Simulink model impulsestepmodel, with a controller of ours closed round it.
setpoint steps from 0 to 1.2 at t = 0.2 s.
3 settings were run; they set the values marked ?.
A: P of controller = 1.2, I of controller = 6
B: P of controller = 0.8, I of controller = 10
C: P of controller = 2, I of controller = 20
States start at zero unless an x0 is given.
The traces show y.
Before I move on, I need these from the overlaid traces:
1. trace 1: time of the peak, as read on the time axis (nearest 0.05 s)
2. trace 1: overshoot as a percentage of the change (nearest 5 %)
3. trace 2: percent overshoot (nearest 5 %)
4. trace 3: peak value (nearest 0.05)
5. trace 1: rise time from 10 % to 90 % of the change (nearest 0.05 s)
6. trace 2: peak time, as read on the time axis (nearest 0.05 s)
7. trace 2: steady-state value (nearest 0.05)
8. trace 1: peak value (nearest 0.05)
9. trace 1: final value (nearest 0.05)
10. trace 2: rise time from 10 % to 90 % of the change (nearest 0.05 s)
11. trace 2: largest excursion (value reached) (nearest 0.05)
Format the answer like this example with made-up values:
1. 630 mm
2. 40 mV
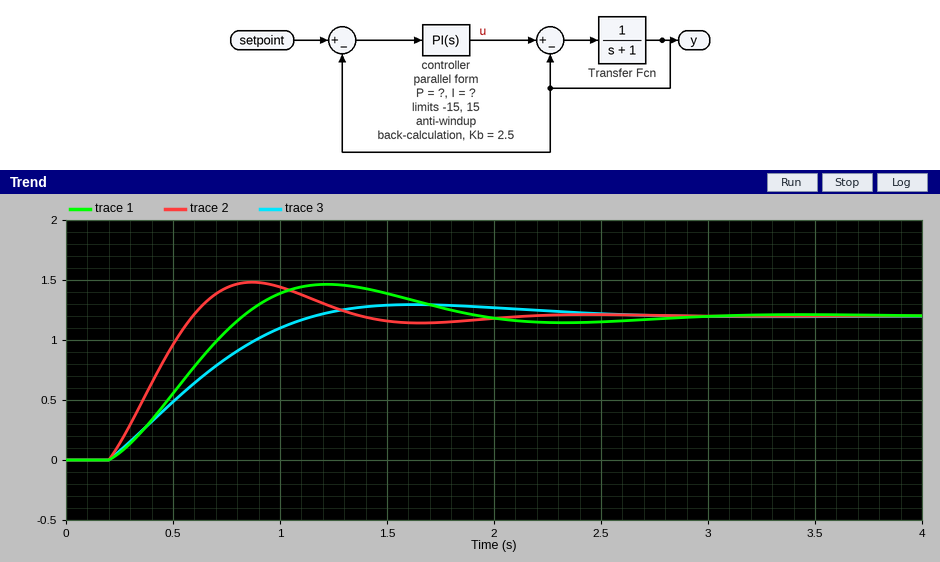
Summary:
1. 1.20 s
2. 20 %
3. 25 %
4. 1.30
5. 0.45 s
6. 0.85 s
7. 1.20
8. 1.45
9. 1.20
10. 0.30 s
11. 1.50
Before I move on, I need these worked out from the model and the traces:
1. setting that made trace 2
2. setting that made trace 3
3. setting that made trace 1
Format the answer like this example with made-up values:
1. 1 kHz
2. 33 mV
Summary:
1. C
2. A
3. B
